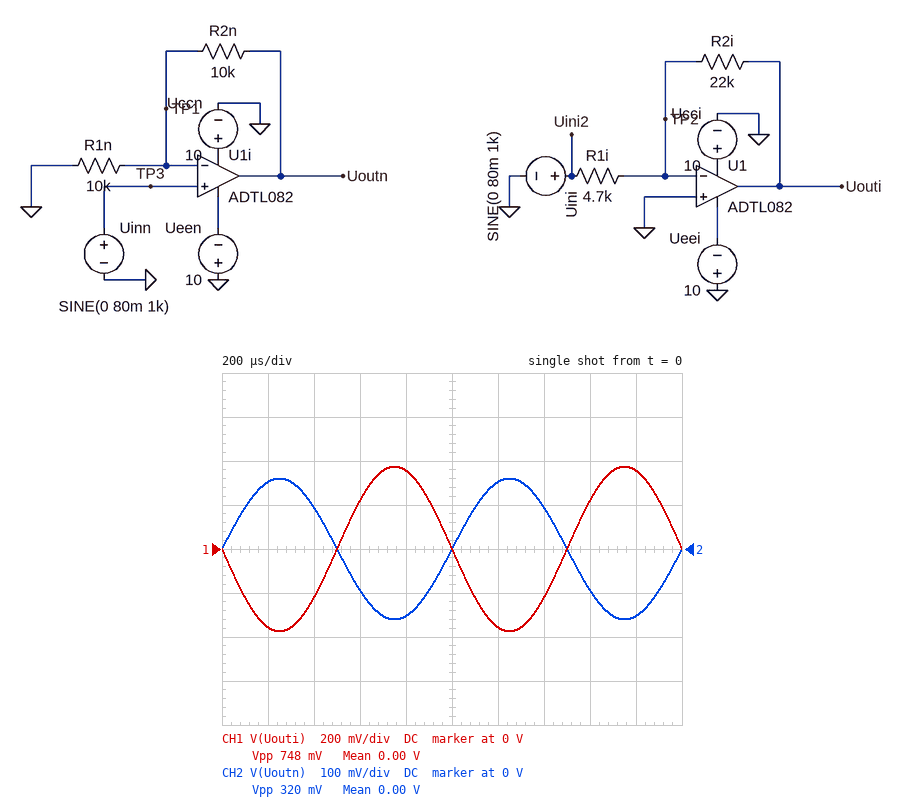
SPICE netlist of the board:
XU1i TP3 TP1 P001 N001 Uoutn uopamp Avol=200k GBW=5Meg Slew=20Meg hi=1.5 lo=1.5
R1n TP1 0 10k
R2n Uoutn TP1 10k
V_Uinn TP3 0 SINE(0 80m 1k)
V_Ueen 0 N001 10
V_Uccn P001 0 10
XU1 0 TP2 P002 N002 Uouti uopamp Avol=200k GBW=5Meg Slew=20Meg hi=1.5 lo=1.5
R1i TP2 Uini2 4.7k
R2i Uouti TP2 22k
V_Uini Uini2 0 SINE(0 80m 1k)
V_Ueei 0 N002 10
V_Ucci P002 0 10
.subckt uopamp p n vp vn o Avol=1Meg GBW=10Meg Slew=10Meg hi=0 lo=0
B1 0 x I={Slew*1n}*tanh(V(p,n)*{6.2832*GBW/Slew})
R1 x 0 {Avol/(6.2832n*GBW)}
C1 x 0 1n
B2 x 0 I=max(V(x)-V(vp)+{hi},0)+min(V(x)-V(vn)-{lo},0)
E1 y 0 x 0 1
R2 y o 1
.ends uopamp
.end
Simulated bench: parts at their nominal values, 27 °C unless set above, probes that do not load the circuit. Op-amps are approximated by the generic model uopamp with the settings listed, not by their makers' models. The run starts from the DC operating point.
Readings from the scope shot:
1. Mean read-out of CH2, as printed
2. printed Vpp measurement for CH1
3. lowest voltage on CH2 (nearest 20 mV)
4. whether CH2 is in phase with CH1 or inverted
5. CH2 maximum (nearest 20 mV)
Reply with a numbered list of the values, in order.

1. 0.00 V
2. 748 mV
3. -160 mV
4. inverted
5. 160 mV
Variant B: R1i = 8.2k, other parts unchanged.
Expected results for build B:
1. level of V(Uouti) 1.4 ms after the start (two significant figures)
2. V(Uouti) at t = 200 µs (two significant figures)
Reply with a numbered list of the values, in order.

1. -130 mV
2. -200 mV
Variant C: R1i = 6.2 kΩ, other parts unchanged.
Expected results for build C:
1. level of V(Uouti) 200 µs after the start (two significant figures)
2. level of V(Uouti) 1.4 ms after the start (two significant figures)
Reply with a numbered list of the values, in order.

1. -270 mV
2. -170 mV
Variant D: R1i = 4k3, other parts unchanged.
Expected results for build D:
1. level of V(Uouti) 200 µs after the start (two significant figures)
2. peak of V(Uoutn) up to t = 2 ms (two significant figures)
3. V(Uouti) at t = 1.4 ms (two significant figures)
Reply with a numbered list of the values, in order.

1. -390 mV
2. 160 mV
3. -240 mV
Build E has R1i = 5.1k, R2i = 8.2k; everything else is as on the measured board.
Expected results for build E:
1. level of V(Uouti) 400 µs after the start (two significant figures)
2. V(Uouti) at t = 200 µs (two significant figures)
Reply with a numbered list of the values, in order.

1. -76 mV
2. -120 mV
